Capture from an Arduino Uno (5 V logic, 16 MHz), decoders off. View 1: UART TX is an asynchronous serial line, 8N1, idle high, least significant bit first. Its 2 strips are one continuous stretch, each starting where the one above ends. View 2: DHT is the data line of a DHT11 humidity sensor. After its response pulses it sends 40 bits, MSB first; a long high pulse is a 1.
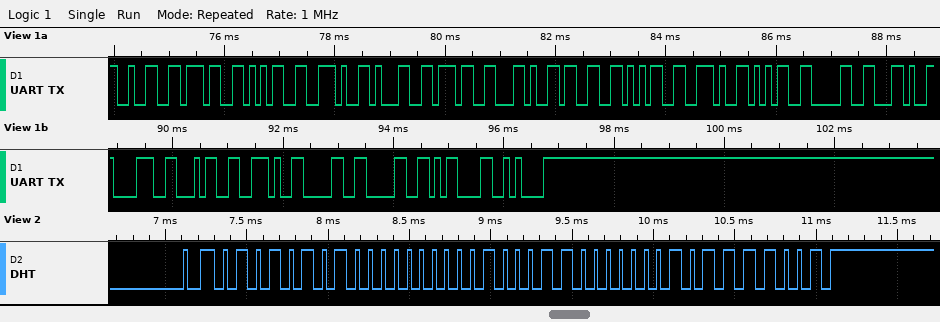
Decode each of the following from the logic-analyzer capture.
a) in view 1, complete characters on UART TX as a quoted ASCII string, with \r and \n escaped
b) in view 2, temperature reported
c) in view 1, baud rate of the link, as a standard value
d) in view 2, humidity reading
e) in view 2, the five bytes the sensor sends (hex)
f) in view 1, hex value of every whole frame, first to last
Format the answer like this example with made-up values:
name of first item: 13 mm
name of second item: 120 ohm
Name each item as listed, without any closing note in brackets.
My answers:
in view 1, complete characters on UART TX as a quoted ASCII string, with \r and \n escaped: "275.17,35.50,84.00\r\n"
in view 2, temperature reported: 35.1 °C
in view 1, baud rate of the link, as a standard value: 9600 baud
in view 2, humidity reading: 85 %
in view 2, the five bytes the sensor sends: 55 00 23 01 79
in view 1, hex value of every whole frame, first to last: 32 37 35 2E 31 37 2C 33 35 2E 35 30 2C 38 34 2E 30 30 0D 0A
